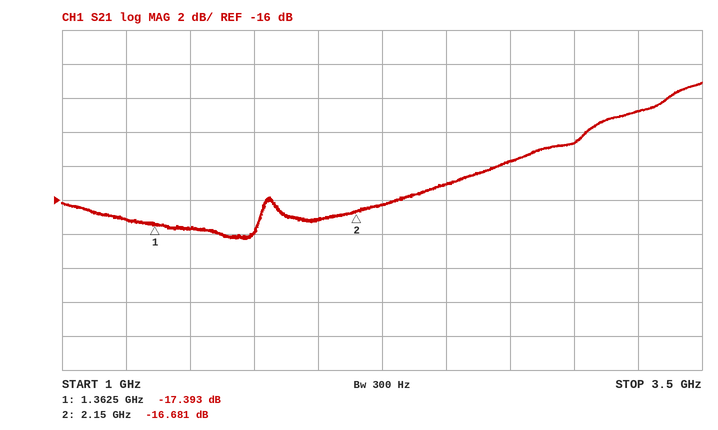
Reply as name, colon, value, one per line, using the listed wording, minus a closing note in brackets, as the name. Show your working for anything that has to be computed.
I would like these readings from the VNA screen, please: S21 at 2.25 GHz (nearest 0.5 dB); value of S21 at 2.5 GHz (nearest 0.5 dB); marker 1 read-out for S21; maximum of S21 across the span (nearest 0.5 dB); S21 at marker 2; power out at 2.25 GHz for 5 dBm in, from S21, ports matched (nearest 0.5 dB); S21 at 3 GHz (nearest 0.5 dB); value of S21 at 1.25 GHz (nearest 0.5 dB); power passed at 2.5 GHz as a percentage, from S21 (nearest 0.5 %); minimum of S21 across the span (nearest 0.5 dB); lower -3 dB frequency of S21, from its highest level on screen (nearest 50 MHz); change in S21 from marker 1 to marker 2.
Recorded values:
S21 at 2.25 GHz: -16.5 dB
value of S21 at 2.5 GHz: -15.0 dB
marker 1 read-out for S21: -17.393 dB
maximum of S21 across the span: -9.0 dB
S21 at marker 2: -16.681 dB
power out at 2.25 GHz for 5 dBm in, from S21, ports matched: 5 dBm + (-16.5 dB) = -11.5 dBm
S21 at 3 GHz: -12.5 dB
value of S21 at 1.25 GHz: -17.0 dB
power passed at 2.5 GHz as a percentage, from S21: 10^(-15/10) ≈ 3.16 %, so 3.0 % to the nearest 0.5 %
minimum of S21 across the span: -18.5 dB
lower -3 dB frequency of S21, from its highest level on screen: 3.05 GHz
change in S21 from marker 1 to marker 2: -16.681 − (-17.393) = 0.712 dB
